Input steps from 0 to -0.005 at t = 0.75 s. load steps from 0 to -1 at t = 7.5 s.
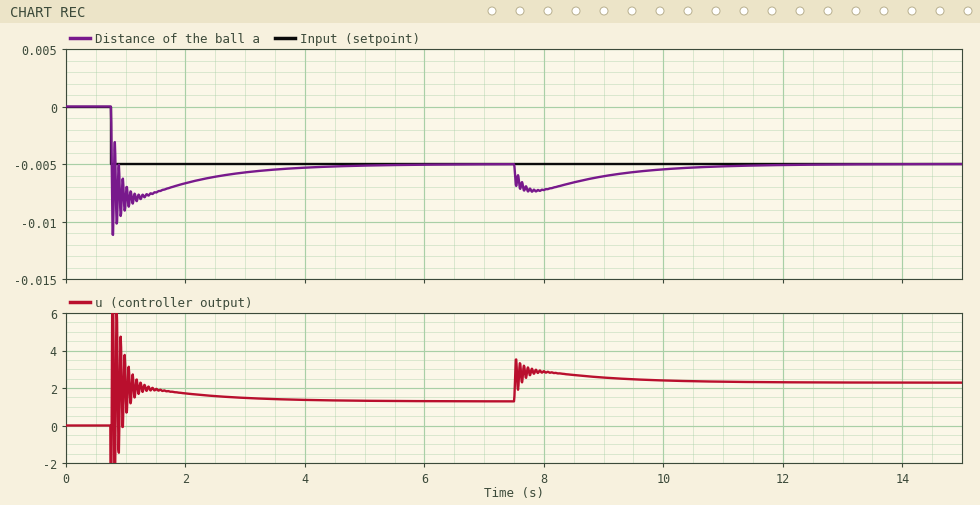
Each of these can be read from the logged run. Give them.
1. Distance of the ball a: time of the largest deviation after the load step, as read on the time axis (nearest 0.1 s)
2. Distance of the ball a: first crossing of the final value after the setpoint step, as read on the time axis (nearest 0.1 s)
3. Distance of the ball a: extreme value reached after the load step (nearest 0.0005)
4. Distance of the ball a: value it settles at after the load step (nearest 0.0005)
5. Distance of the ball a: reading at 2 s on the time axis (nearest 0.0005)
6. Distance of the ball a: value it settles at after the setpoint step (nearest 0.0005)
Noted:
7.8 s
0.8 s
-0.0075
-0.0050
-0.0065
-0.0050
